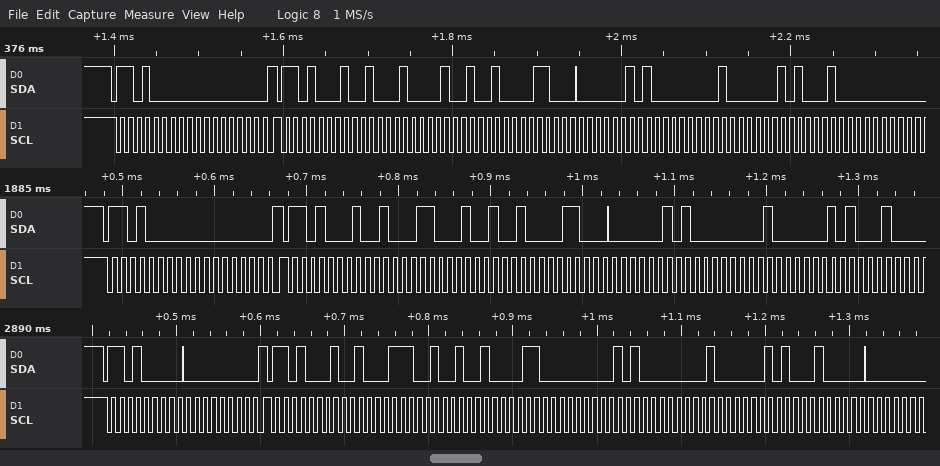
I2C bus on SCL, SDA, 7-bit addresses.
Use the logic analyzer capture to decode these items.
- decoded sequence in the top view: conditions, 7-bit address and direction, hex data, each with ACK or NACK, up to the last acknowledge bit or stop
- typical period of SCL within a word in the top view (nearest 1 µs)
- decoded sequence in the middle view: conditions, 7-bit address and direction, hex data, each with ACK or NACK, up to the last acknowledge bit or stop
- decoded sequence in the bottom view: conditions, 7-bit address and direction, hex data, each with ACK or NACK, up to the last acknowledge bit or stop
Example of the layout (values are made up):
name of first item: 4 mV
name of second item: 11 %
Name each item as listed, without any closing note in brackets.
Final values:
decoded sequence in the top view: conditions, 7-bit address and direction, hex data, each with ACK or NACK, up to the last acknowledge bit or stop: start, address 68 write ACK, 00 ACK, repeated start, address 68 read ACK, 44 ACK, 49 ACK, 18 ACK, 05 ACK, 01 ACK, 05 ACK, 20 ACK
typical period of SCL within a word in the top view: 10 µs
decoded sequence in the middle view: conditions, 7-bit address and direction, hex data, each with ACK or NACK, up to the last acknowledge bit or stop: start, address 68 write ACK, 00 ACK, repeated start, address 68 read ACK, 46 ACK, 49 ACK, 18 ACK, 05 ACK, 01 ACK, 05 ACK
decoded sequence in the bottom view: conditions, 7-bit address and direction, hex data, each with ACK or NACK, up to the last acknowledge bit or stop: start, address 68 write ACK, 00 ACK, repeated start, address 68 read ACK, 47 ACK, 49 ACK, 18 ACK, 05 ACK, 01 ACK, 05 ACK, 20 ACK
